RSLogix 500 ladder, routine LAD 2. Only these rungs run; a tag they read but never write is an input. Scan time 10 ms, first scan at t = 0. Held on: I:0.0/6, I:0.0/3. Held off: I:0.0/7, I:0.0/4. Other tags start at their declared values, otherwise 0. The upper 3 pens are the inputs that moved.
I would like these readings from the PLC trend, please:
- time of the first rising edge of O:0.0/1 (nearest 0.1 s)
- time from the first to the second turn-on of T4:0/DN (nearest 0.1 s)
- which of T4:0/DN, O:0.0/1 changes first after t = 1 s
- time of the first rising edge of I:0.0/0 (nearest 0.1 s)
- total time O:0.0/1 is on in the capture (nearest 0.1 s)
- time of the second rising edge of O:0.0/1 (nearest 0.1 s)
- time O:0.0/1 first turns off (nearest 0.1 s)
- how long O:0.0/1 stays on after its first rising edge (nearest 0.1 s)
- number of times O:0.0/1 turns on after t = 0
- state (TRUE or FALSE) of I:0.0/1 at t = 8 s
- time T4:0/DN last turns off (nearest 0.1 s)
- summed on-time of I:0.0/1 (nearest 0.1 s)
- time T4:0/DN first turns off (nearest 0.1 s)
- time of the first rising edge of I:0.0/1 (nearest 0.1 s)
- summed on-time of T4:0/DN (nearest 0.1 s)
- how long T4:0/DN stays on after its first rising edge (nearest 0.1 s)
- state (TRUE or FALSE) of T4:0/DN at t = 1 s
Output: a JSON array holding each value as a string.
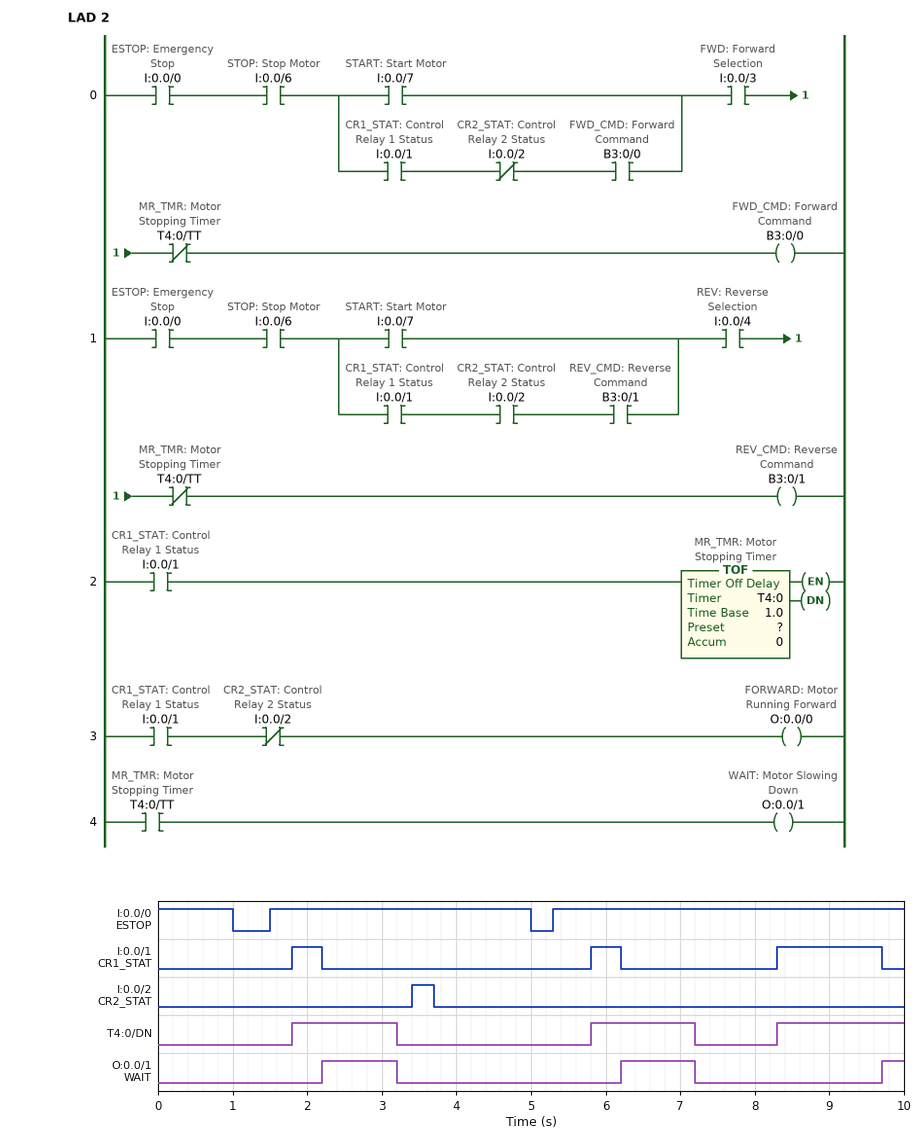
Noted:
["2.2 s", "4.0 s", "T4:0/DN", "1.5 s", "2.3 s", "6.2 s", "3.2 s", "1.0 s", "3", "FALSE", "7.2 s", "2.2 s", "3.2 s", "1.8 s", "4.5 s", "1.4 s", "FALSE"]
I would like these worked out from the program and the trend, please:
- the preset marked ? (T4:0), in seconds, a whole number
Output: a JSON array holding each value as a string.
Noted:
["1 s"]
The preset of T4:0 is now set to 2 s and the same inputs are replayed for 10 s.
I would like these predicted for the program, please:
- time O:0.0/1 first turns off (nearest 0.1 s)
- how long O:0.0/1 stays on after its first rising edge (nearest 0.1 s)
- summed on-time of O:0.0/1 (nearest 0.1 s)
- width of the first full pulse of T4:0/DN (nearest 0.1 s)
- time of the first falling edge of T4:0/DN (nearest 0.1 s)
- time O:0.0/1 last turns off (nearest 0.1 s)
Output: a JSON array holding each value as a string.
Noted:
["4.2 s", "2.0 s", "4.3 s", "2.4 s", "4.2 s", "8.2 s"]
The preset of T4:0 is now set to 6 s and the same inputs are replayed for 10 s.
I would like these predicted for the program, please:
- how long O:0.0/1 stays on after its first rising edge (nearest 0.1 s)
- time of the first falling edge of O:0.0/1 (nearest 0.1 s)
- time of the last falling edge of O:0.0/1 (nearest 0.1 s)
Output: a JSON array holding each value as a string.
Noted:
["3.6 s", "5.8 s", "8.3 s"]
